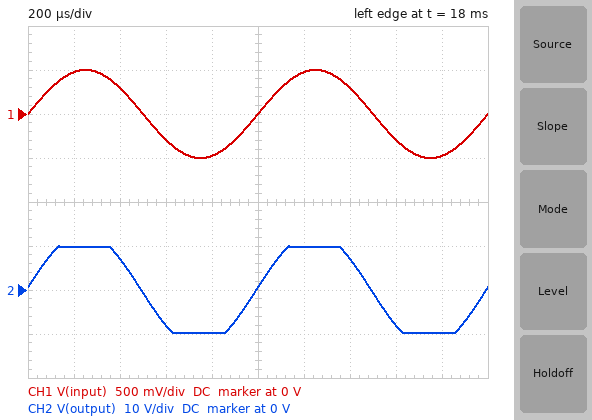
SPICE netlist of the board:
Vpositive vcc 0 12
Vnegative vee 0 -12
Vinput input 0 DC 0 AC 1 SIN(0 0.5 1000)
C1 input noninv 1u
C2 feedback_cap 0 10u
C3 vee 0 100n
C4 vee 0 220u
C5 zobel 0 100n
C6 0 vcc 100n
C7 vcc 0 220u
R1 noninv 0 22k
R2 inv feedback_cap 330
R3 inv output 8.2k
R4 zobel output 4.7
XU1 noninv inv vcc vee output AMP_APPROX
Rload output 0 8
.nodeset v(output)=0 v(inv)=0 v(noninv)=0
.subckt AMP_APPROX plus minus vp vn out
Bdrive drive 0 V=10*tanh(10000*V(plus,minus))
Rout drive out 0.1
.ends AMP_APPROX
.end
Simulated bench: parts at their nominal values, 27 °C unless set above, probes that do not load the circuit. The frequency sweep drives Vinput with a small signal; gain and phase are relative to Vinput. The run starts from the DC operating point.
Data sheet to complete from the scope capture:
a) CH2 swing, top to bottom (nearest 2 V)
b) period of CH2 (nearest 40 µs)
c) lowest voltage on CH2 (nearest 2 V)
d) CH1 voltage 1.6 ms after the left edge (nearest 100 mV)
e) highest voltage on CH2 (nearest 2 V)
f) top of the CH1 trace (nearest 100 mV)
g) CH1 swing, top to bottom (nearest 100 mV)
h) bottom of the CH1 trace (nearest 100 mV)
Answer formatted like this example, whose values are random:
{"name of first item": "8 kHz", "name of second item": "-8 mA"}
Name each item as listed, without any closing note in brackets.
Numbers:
{"CH2 swing, top to bottom": "20 V", "period of CH2": "1.00 ms", "lowest voltage on CH2": "-10 V", "CH1 voltage 1.6 ms after the left edge": "-300 mV", "highest voltage on CH2": "10 V", "top of the CH1 trace": "500 mV", "CH1 swing, top to bottom": "1.0 V", "bottom of the CH1 trace": "-500 mV"}
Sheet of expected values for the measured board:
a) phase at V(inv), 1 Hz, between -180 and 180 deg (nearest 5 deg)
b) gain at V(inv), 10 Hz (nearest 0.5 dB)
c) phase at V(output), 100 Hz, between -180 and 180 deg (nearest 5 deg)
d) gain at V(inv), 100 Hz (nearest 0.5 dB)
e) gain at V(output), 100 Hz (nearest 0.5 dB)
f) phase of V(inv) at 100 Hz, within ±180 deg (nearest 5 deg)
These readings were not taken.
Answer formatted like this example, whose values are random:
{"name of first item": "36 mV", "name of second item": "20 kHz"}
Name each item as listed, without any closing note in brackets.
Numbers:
{"phase at V(inv), 1 Hz, between -180 and 180 deg": "80 deg", "gain at V(inv), 10 Hz": "-2.0 dB", "phase at V(output), 100 Hz, between -180 and 180 deg": "30 deg", "gain at V(inv), 100 Hz": "0 dB", "gain at V(output), 100 Hz": "27.5 dB", "phase of V(inv) at 100 Hz, within ±180 deg": "5 deg"}
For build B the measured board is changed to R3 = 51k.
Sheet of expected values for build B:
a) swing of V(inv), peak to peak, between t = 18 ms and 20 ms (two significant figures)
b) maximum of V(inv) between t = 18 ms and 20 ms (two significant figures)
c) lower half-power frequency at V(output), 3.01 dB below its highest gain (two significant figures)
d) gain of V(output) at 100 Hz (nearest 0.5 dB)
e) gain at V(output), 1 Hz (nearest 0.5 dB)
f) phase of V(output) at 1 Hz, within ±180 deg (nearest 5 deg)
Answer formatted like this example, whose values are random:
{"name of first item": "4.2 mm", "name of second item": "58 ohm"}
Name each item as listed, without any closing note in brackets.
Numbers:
{"swing of V(inv), peak to peak, between t = 18 ms and 20 ms": "140 mV", "maximum of V(inv) between t = 18 ms and 20 ms": "70 mV", "lower half-power frequency at V(output), 3.01 dB below its highest gain": "49 Hz", "gain of V(output) at 100 Hz": "43.0 dB", "gain at V(output), 1 Hz": "-6.5 dB", "phase of V(output) at 1 Hz, within ±180 deg": "155 deg"}
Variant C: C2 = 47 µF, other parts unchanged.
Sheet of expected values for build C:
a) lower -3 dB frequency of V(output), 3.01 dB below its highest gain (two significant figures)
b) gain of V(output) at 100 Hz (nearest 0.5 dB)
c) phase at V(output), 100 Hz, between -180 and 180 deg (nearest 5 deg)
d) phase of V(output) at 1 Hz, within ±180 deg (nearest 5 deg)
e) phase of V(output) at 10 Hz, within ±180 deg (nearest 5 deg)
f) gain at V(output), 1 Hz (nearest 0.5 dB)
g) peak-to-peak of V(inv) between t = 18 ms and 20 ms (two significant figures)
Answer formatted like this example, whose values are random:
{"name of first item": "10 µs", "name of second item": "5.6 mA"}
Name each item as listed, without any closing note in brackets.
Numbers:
{"lower -3 dB frequency of V(output), 3.01 dB below its highest gain": "14 Hz", "gain of V(output) at 100 Hz": "28.0 dB", "phase at V(output), 100 Hz, between -180 and 180 deg": "10 deg", "phase of V(output) at 1 Hz, within ±180 deg": "145 deg", "phase of V(output) at 10 Hz, within ±180 deg": "80 deg", "gain at V(output), 1 Hz": "-8.5 dB", "peak-to-peak of V(inv) between t = 18 ms and 20 ms": "770 mV"}
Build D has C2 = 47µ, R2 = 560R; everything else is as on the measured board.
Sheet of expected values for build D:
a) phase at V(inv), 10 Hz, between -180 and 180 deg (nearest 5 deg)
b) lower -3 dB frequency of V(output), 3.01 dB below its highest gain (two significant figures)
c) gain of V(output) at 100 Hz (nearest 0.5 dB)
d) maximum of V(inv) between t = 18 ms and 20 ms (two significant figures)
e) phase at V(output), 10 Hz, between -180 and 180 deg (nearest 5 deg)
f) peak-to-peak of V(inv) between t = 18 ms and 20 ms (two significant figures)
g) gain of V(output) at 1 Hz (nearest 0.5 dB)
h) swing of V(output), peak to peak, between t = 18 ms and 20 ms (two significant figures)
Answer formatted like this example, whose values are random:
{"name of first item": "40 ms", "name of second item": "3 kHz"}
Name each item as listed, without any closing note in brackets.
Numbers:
{"phase at V(inv), 10 Hz, between -180 and 180 deg": "35 deg", "lower -3 dB frequency of V(output), 3.01 dB below its highest gain": "10 Hz", "gain of V(output) at 100 Hz": "24.0 dB", "maximum of V(inv) between t = 18 ms and 20 ms": "500 mV", "phase at V(output), 10 Hz, between -180 and 180 deg": "65 deg", "peak-to-peak of V(inv) between t = 18 ms and 20 ms": "1.0 V", "gain of V(output) at 1 Hz": "-8.5 dB", "swing of V(output), peak to peak, between t = 18 ms and 20 ms": "16 V"}
